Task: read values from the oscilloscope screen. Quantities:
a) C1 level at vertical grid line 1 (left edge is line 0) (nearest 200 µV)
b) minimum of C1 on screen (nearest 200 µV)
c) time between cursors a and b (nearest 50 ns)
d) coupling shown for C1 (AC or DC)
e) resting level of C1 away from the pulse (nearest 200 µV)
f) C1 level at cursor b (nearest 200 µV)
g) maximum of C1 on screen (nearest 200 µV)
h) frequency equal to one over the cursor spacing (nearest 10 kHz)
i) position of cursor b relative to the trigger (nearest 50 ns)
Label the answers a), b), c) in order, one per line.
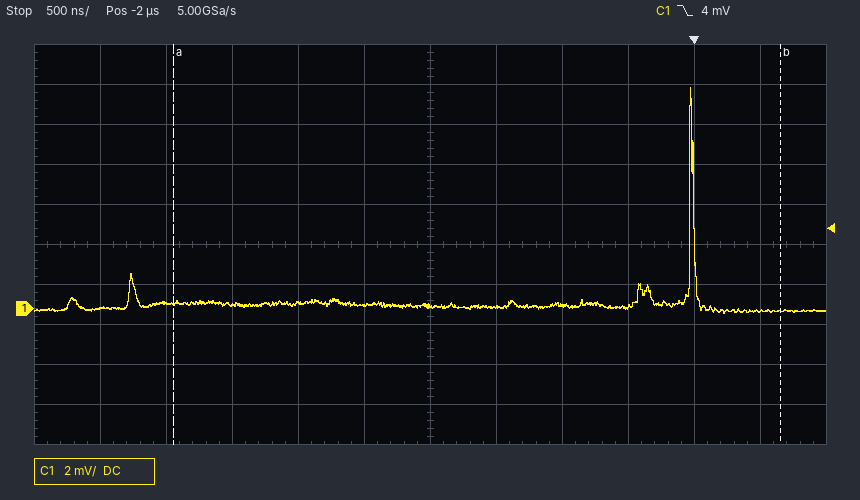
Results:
a) 0.0 mV
b) -200 µV
c) 4.60 µs
d) DC
e) 200 µV
f) -200 µV
g) 11.0 mV
h) 220 kHz
i) +650 ns
